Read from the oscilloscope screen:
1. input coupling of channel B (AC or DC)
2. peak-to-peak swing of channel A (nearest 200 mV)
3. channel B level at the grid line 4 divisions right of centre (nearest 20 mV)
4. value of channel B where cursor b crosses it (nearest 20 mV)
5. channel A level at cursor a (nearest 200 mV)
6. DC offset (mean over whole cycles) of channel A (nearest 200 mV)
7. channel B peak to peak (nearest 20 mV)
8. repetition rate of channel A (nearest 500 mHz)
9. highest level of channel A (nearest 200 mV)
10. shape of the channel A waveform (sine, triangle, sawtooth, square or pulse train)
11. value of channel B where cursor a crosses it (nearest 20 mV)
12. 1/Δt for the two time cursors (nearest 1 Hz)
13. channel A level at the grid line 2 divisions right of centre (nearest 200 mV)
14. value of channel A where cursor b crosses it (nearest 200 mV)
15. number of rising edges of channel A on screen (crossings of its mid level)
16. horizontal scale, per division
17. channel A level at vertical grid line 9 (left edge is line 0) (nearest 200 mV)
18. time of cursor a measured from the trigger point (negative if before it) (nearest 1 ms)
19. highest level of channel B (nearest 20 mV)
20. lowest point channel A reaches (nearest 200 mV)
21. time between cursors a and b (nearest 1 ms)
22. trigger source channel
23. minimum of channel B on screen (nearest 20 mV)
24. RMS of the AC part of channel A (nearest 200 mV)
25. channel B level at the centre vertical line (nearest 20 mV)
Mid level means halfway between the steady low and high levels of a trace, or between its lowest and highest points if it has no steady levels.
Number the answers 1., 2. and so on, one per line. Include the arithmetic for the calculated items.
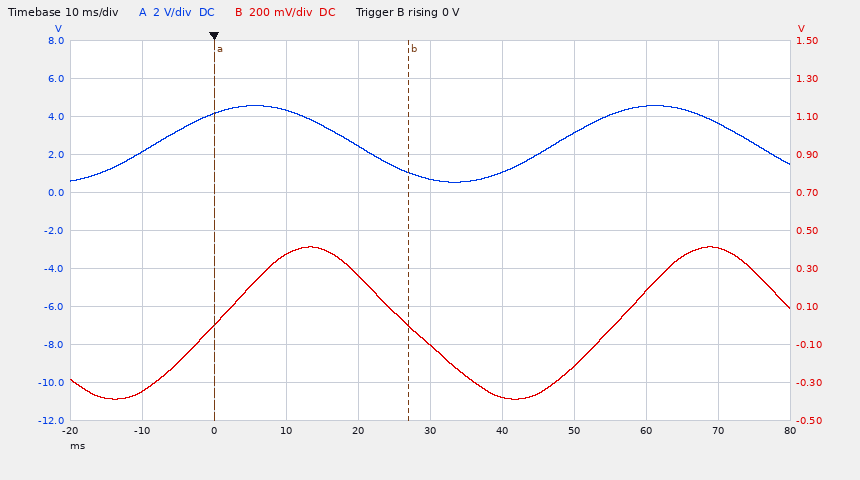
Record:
1. DC
2. 4.6 V − (600 mV) = 4.0 V
3. 400 mV
4. 0 mV
5. 4.2 V
6. (4.6 V + (600 mV)) / 2 ≈ 2.6 V
7. 420 mV − (-380 mV) = 800 mV
8. 18.0 Hz
9. 4.6 V
10. sine
11. 0 mV
12. 1 / 27 ms ≈ 37 Hz
13. 3.2 V
14. 1.0 V
15. 2
16. 10 ms
17. 3.6 V
18. 0 ms
19. 420 mV
20. 600 mV
21. 27 ms
22. channel B
23. -380 mV
24. 4.0 V / (2√2) ≈ 1.4 V
25. -100 mV
